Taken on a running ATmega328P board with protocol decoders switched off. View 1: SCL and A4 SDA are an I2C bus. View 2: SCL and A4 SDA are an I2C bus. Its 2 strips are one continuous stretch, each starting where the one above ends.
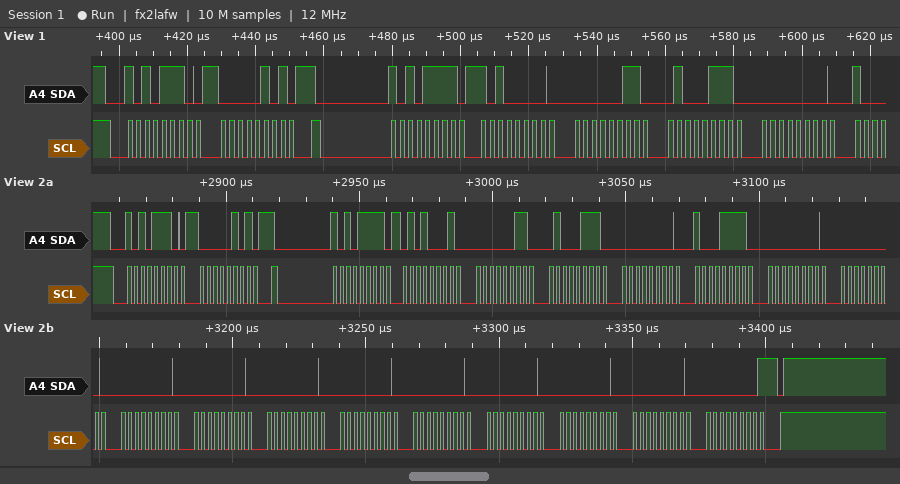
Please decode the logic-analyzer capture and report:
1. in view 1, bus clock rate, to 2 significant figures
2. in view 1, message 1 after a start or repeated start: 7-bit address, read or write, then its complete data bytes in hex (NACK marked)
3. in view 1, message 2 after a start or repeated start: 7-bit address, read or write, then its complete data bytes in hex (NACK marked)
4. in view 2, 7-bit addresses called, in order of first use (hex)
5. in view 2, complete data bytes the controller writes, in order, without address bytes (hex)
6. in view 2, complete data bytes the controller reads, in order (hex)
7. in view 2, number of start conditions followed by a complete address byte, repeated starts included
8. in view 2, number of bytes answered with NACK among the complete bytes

400 kHz
0x57 write: 05
0x57 read: A0 03 47 00
0x57
05
51 03 47 00 8F 00 00 00 00 00 00 00 00 00 00 00
2
1
